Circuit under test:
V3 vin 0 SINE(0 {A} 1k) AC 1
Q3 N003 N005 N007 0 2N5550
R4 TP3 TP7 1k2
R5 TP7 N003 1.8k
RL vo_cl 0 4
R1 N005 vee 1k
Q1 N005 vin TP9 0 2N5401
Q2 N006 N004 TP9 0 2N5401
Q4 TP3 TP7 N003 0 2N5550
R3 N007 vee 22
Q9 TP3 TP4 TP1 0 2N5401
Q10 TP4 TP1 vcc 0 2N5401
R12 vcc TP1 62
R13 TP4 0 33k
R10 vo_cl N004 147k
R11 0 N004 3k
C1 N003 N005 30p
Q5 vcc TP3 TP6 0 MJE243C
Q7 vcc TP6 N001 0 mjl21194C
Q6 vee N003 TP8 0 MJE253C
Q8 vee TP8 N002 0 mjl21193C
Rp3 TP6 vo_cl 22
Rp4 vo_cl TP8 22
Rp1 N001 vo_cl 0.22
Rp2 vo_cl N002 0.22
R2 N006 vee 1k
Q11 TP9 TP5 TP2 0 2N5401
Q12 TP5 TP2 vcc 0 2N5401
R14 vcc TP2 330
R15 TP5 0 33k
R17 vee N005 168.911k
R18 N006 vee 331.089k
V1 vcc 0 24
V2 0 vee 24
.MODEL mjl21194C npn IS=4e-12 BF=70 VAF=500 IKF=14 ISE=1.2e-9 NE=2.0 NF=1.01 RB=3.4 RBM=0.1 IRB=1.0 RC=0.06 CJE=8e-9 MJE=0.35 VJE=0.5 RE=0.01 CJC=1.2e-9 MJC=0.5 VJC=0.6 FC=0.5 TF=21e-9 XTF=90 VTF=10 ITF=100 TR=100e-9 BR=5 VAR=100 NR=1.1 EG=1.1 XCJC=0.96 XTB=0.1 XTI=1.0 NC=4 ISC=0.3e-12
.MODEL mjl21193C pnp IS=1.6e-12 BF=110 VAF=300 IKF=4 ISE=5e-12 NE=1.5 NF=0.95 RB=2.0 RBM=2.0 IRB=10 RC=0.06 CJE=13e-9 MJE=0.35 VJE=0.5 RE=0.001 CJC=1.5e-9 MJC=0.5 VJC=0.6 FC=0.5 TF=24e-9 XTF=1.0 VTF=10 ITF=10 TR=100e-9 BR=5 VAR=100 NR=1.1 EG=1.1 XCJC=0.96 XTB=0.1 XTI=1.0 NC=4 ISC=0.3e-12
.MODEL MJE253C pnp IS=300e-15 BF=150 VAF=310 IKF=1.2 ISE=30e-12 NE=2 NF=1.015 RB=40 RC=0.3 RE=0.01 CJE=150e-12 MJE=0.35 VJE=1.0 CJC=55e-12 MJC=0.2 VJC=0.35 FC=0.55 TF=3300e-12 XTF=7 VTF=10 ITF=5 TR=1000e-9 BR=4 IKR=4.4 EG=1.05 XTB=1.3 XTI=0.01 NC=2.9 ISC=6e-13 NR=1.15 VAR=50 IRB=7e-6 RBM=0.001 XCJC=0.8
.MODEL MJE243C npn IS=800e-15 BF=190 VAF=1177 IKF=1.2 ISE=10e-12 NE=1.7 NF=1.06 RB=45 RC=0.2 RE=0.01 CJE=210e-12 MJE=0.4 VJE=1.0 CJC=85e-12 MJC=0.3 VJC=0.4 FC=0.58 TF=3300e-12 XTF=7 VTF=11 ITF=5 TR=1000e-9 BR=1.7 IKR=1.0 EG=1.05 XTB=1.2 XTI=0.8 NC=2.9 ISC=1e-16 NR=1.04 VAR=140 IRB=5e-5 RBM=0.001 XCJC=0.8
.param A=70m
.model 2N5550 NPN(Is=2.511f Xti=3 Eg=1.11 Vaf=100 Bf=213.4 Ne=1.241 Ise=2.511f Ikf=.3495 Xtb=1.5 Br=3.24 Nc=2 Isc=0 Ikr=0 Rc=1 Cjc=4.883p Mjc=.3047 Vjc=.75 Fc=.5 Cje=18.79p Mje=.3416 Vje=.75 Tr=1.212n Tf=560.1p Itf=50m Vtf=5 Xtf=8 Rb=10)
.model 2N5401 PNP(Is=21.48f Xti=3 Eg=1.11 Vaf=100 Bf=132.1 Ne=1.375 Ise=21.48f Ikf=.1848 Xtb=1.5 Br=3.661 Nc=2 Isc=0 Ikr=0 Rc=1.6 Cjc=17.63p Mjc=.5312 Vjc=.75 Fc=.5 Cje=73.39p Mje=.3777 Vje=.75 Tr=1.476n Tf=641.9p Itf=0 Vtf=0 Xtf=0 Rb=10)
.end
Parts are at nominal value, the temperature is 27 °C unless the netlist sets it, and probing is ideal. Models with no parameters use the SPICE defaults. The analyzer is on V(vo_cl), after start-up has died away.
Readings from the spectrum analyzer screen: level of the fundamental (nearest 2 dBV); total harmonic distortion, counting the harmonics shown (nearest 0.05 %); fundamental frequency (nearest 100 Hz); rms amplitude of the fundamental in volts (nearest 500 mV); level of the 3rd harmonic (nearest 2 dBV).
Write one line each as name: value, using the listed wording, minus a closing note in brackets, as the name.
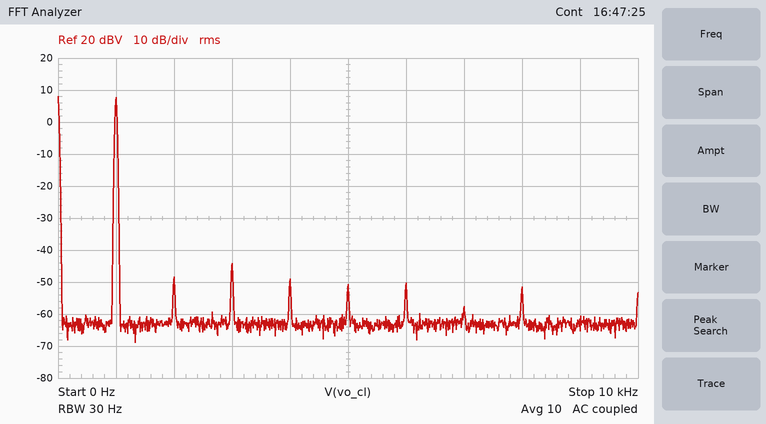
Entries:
level of the fundamental: 8 dBV
total harmonic distortion, counting the harmonics shown: 0.25 %
fundamental frequency: 1.0 kHz
rms amplitude of the fundamental in volts: 2.5 V
level of the 3rd harmonic: -44 dBV
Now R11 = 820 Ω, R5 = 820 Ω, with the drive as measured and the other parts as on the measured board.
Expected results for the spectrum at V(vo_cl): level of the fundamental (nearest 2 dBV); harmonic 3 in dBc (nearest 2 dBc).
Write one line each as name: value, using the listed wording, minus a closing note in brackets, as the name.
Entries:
level of the fundamental: 18 dBV
harmonic 3 in dBc: -56 dBc
